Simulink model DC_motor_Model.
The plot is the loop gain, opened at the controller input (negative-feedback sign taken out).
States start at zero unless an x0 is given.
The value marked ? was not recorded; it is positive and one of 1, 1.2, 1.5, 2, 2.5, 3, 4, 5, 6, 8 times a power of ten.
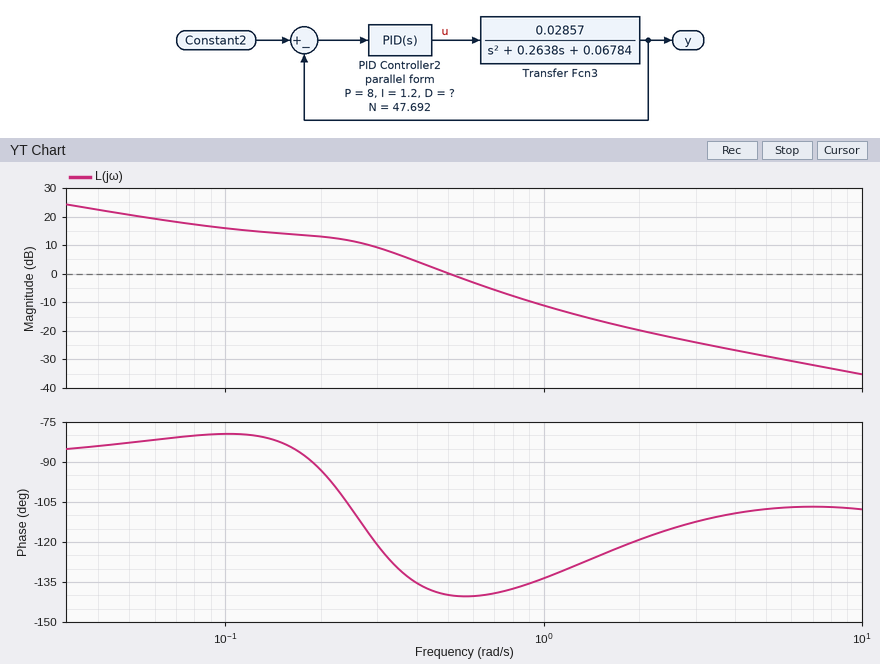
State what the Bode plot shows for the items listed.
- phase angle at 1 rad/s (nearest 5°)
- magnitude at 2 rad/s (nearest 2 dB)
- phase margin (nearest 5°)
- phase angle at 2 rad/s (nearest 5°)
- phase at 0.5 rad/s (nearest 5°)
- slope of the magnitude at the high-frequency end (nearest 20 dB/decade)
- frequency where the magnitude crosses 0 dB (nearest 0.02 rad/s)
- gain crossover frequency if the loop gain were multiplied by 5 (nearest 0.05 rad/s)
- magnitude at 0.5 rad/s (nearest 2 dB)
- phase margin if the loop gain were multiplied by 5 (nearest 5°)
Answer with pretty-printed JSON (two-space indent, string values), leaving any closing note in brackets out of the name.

{
  "phase angle at 1 rad/s": "-135°",
  "magnitude at 2 rad/s": "-20 dB",
  "phase margin": "40°",
  "phase angle at 2 rad/s": "-120°",
  "phase at 0.5 rad/s": "-140°",
  "slope of the magnitude at the high-frequency end": "-20 dB/decade",
  "frequency where the magnitude crosses 0 dB": "0.50 rad/s",
  "gain crossover frequency if the loop gain were multiplied by 5": "1.25 rad/s",
  "magnitude at 0.5 rad/s": "0 dB",
  "phase margin if the loop gain were multiplied by 5": "50°"
}
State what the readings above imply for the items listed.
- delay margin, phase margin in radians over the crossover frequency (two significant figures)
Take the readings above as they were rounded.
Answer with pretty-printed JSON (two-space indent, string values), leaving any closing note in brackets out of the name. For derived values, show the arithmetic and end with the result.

{
  "delay margin, phase margin in radians over the crossover frequency": "40 × π / 180 / 0.5 = 1.4 s"
}
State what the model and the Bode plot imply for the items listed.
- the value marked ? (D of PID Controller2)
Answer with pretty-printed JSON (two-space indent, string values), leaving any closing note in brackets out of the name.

{
  "the value marked ?": "6"
}
